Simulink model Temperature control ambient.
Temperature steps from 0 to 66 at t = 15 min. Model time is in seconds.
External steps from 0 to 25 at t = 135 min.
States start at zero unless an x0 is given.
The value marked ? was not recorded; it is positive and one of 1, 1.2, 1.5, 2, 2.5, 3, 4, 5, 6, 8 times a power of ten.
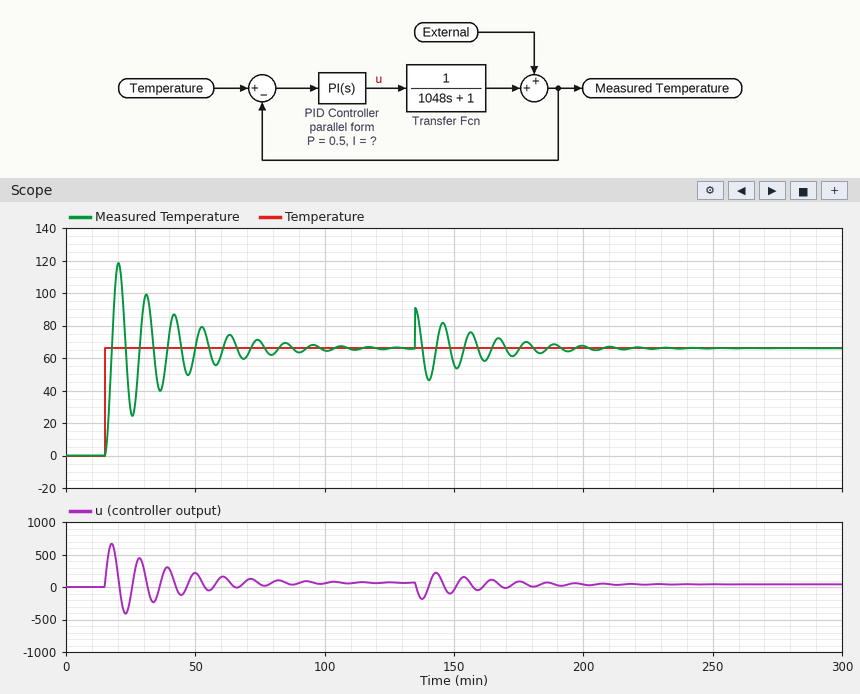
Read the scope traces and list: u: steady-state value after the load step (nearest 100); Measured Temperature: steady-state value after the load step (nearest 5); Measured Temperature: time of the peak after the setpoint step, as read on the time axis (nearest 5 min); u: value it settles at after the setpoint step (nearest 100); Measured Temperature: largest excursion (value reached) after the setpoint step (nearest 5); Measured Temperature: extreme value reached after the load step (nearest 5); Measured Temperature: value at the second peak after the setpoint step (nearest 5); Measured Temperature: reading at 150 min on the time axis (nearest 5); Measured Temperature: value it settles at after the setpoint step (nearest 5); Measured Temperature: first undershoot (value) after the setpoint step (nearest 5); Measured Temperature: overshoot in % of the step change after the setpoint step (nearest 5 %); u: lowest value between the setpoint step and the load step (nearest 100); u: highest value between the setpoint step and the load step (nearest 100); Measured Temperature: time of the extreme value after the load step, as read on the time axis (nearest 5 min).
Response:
0
65
20 min
100
120
90
100
55
65
25
80 %
-400
700
135 min
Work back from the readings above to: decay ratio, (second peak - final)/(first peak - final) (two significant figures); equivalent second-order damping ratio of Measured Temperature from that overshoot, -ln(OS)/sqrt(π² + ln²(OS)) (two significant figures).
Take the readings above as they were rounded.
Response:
0.64
0.071
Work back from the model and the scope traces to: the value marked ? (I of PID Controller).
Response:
0.1
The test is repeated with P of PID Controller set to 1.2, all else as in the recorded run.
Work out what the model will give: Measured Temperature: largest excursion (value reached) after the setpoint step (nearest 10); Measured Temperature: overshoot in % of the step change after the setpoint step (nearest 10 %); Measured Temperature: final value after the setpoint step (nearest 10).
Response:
110
70 %
70
